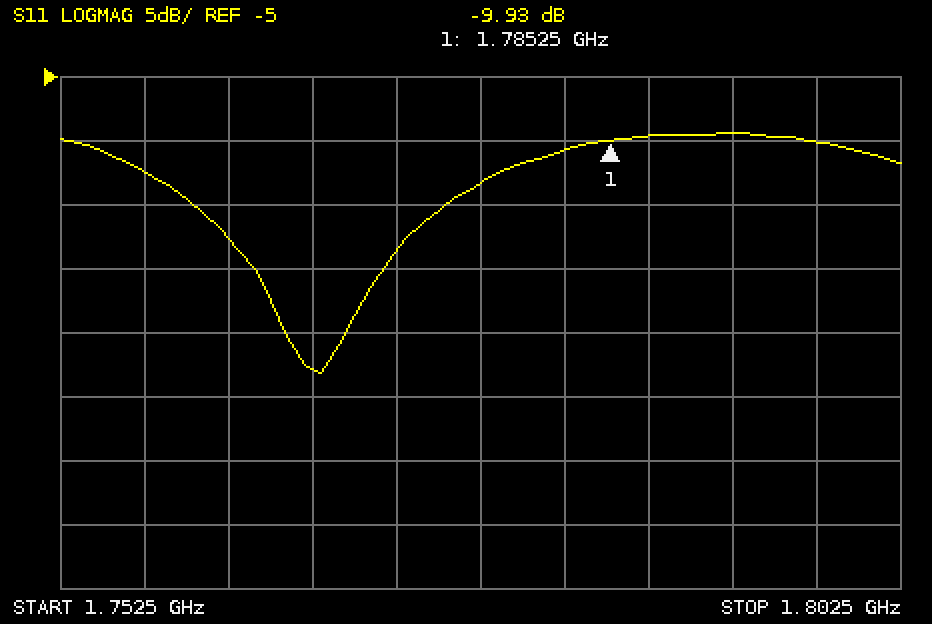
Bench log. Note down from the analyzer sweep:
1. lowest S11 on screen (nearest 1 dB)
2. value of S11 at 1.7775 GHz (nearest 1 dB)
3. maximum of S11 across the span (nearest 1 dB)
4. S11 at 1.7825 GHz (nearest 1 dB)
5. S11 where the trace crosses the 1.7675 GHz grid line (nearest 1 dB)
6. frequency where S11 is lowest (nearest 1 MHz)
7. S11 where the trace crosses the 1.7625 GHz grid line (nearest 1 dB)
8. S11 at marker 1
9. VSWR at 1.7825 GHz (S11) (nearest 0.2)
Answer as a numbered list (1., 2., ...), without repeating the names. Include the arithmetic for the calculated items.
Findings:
1. -28 dB
2. -13 dB
3. -9 dB
4. -11 dB
5. -28 dB
6. 1.768 GHz
7. -18 dB
8. -9.93 dB
9. |Γ| = 10^(-11/20) = 0.2818; VSWR = (1 + 0.2818)/(1 − 0.2818) ≈ 1.8
